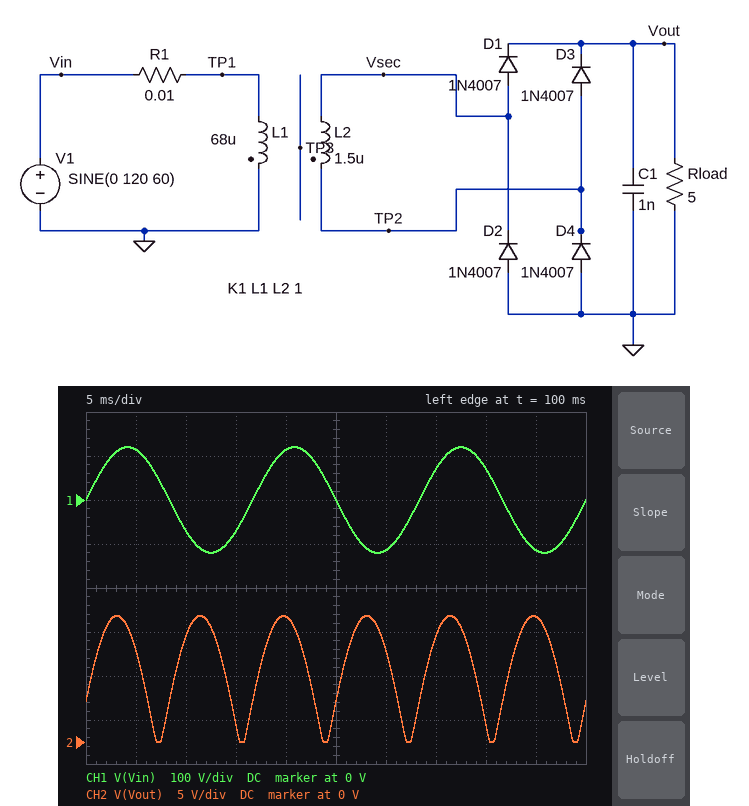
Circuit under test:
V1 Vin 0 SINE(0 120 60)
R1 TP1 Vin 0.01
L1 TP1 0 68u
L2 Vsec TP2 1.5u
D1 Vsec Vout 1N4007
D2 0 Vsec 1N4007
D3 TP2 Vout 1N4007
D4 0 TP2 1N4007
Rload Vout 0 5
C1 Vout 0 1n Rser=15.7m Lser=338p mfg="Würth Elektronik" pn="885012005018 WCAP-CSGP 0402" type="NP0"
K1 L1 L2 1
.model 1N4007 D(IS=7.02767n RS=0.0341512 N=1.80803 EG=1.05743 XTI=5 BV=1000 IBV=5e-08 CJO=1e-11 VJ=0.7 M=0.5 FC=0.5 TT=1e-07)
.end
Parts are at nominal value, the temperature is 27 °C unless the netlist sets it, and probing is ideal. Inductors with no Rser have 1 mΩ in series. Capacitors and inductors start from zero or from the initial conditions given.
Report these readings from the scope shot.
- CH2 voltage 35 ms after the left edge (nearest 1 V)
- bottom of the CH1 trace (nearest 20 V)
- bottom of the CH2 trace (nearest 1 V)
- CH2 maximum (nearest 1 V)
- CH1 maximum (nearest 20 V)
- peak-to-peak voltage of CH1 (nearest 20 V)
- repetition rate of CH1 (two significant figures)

12 V
-120 V
0 V
14 V
120 V
240 V
60 Hz
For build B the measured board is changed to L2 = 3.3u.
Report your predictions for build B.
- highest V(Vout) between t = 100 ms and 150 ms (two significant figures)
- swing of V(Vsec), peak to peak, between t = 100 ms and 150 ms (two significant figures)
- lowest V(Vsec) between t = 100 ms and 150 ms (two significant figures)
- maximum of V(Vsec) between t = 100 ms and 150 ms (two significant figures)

22 V
24 V
-1.1 V
23 V
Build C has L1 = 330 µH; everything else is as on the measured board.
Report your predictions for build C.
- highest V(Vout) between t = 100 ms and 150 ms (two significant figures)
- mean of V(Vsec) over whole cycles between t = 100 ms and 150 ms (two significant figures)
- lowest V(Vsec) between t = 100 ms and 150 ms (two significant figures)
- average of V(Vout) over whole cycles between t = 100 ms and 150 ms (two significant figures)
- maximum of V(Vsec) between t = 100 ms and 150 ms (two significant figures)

6.2 V
1.7 V
-930 mV
3.5 V
7.1 V
